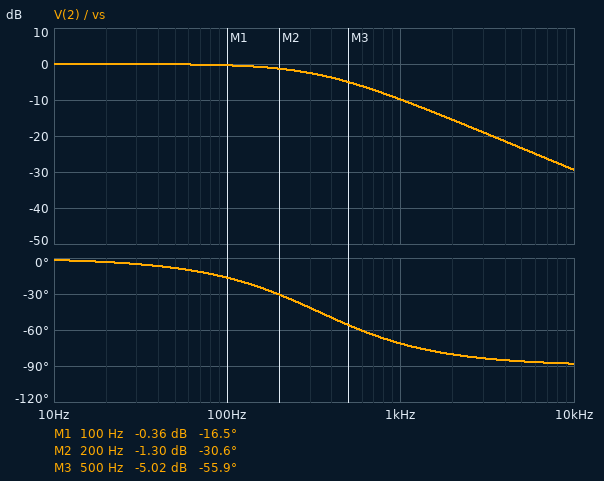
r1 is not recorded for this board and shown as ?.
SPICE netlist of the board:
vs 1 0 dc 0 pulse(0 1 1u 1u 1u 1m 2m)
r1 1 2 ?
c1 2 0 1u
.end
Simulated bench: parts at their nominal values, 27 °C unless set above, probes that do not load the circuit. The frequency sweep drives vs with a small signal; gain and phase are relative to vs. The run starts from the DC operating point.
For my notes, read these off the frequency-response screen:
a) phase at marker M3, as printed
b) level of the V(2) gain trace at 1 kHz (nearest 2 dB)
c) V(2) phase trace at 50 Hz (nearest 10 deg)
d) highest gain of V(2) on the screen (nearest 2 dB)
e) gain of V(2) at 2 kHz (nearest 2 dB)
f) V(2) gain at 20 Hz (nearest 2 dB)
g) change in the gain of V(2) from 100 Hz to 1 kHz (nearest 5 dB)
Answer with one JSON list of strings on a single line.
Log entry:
["-55.9 deg", "-10 dB", "-10 deg", "0 dB", "-16 dB", "0 dB", "-10 dB"]
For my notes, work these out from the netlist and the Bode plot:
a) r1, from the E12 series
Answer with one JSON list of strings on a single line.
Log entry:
["470 Ω"]
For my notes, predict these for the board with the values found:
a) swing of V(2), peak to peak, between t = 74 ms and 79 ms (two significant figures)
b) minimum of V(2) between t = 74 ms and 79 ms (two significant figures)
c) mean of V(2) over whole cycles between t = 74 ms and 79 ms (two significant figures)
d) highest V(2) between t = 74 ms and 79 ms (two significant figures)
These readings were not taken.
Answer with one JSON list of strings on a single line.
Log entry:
["790 mV", "110 mV", "500 mV", "890 mV"]
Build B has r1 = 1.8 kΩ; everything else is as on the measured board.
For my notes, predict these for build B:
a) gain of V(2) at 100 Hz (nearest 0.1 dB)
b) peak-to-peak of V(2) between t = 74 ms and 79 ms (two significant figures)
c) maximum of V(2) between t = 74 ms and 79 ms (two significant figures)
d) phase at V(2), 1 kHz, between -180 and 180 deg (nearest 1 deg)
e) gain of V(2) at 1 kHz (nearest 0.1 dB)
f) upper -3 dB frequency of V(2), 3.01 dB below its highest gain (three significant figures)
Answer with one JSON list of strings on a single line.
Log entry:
["-3.6 dB", "270 mV", "640 mV", "-85 deg", "-21.1 dB", "88.4 Hz"]
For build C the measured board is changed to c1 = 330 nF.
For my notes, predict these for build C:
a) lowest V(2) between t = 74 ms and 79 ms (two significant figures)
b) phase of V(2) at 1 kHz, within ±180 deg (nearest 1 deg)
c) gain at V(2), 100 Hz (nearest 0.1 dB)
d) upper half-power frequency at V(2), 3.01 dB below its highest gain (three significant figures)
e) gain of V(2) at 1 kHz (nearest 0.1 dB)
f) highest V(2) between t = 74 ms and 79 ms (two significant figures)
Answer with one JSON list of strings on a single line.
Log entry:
["1.6 mV", "-44 deg", "0 dB", "1.03 kHz", "-2.9 dB", "1.0 V"]
